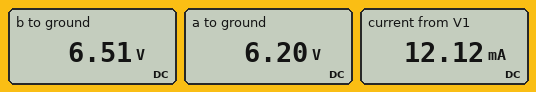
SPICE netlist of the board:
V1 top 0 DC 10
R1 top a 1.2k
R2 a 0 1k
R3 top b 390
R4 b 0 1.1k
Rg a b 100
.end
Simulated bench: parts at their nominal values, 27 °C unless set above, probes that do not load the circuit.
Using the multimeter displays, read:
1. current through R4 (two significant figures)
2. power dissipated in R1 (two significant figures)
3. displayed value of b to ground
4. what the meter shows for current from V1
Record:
5.9 mA
12 mW
6.51 V
12.12 mA
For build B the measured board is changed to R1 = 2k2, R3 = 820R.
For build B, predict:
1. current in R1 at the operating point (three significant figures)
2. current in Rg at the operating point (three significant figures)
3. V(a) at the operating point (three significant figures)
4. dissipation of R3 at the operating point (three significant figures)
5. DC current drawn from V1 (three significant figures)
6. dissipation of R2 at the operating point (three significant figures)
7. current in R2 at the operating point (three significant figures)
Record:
2.48 mA
2.07 mA
4.55 V
33.5 mW
8.87 mA
20.7 mW
4.55 mA
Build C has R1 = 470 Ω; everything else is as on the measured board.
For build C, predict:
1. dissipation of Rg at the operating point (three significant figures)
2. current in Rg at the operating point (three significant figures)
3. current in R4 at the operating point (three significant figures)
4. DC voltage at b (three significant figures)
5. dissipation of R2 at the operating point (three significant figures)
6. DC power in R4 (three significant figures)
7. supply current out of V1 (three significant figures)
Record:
67.1 µW
819 µA
6.50 mA
7.15 V
49.9 mW
46.4 mW
13.6 mA
